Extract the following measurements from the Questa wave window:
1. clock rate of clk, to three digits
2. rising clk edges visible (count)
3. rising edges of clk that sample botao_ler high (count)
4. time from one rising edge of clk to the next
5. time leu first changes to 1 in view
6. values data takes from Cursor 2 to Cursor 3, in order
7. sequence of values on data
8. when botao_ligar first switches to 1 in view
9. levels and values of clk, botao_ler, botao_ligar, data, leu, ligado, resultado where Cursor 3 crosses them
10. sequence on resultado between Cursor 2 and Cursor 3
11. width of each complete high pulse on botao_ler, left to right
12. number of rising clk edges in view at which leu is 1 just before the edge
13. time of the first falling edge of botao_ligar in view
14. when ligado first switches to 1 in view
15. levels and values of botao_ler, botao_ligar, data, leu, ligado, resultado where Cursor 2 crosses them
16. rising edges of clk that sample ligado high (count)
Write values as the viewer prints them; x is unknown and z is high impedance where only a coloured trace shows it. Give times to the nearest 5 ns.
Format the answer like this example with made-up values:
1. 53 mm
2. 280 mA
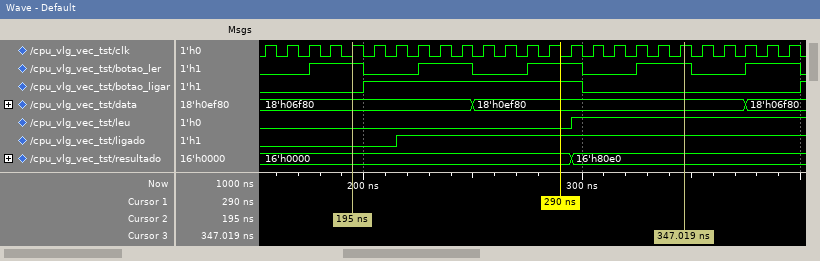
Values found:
1. 100 MHz
2. 25
3. 10
4. 10 ns
5. 295 ns
6. 18'h06f80, 18'h0ef80
7. 18'h06f80, 18'h0ef80, 18'h06f80
8. 200 ns
9. clk=1, botao_ler=1, botao_ligar=0, data=18'h0ef80, leu=1, ligado=1, resultado=16'h80e0
10. 16'h0000, 16'h80e0
11. 25 ns, 25 ns, 25 ns, 25 ns, 25 ns
12. 10
13. 300 ns
14. 215 ns
15. botao_ler=1, botao_ligar=0, data=18'h06f80, leu=0, ligado=0, resultado=16'h0000
16. 18
